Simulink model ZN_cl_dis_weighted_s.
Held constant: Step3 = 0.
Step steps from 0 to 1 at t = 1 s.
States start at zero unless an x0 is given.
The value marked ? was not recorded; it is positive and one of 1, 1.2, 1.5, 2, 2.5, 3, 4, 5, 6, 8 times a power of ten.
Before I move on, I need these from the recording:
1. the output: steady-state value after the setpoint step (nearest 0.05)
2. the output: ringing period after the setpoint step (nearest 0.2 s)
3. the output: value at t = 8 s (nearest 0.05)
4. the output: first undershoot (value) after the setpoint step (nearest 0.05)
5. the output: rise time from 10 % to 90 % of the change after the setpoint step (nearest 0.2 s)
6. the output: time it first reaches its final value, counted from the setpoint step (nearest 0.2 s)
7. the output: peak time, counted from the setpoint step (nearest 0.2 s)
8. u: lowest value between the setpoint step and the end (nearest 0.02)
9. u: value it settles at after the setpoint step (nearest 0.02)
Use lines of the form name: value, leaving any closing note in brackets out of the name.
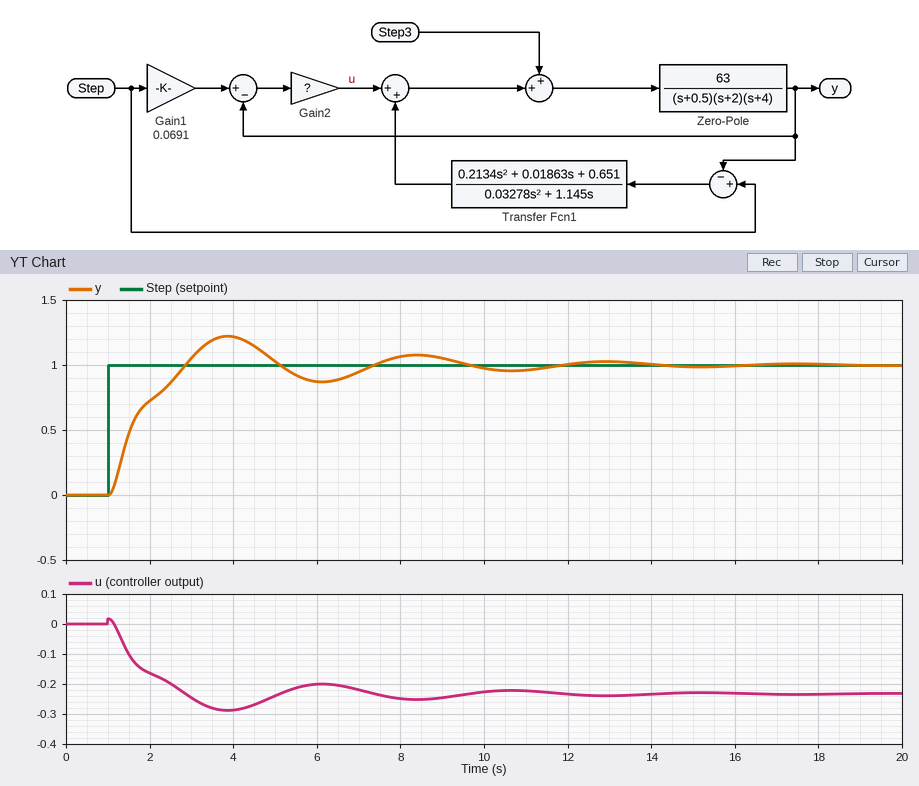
the output: steady-state value after the setpoint step: 1.00
the output: ringing period after the setpoint step: 4.6 s
the output: value at t = 8 s: 1.05
the output: first undershoot (value) after the setpoint step: 0.85
the output: rise time from 10 % to 90 % of the change after the setpoint step: 1.4 s
the output: time it first reaches its final value, counted from the setpoint step: 1.8 s
the output: peak time, counted from the setpoint step: 2.8 s
u: lowest value between the setpoint step and the end: -0.28
u: value it settles at after the setpoint step: -0.24
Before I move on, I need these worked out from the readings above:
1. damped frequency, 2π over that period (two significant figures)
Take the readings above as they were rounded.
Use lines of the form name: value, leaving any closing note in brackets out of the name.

damped frequency, 2π over that period: 1.4 rad/s
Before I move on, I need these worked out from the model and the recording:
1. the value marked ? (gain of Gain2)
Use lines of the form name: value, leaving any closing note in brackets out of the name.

the value marked ?: 0.25
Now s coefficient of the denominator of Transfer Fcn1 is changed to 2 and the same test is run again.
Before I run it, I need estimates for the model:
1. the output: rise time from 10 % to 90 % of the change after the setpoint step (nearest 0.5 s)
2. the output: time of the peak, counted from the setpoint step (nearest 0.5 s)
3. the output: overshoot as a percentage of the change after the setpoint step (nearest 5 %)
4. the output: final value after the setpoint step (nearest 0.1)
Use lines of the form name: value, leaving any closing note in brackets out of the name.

the output: rise time from 10 % to 90 % of the change after the setpoint step: 2.0 s
the output: time of the peak, counted from the setpoint step: 3.5 s
the output: overshoot as a percentage of the change after the setpoint step: 15 %
the output: final value after the setpoint step: 1.0
